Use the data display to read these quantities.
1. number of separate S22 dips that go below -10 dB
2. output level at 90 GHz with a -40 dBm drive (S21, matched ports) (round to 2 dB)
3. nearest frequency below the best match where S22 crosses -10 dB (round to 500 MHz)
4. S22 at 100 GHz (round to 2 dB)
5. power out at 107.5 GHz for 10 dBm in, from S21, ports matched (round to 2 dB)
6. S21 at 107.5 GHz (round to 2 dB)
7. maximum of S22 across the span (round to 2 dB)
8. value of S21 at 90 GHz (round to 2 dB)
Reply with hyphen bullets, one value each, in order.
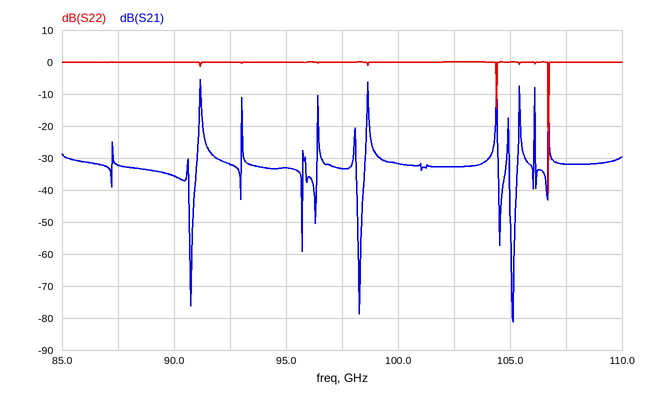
- 2
- -76 dBm
- 106.5 GHz
- 0 dB
- -22 dBm
- -32 dB
- 0 dB
- -36 dB
